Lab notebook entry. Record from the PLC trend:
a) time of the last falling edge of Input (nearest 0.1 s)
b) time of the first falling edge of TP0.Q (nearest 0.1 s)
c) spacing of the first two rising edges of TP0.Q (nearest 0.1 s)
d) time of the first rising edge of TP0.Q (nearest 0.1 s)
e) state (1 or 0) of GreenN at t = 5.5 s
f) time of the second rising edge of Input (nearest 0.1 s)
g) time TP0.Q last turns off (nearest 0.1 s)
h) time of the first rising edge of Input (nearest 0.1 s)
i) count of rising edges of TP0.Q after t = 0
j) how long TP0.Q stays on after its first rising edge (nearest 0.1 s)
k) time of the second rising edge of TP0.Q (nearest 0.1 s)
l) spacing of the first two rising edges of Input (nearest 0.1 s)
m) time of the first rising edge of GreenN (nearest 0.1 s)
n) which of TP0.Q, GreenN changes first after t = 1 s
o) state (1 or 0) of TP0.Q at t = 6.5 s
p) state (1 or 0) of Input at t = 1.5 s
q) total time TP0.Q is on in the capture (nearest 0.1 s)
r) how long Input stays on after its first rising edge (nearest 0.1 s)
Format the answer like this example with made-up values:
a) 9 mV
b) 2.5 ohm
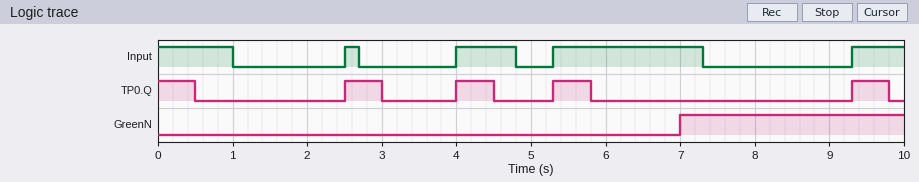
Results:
a) 7.3 s
b) 0.5 s
c) 1.5 s
d) 2.5 s
e) 0
f) 4.0 s
g) 9.8 s
h) 2.5 s
i) 4
j) 0.5 s
k) 4.0 s
l) 1.5 s
m) 7.0 s
n) TP0.Q
o) 0
p) 0
q) 2.5 s
r) 0.2 s
